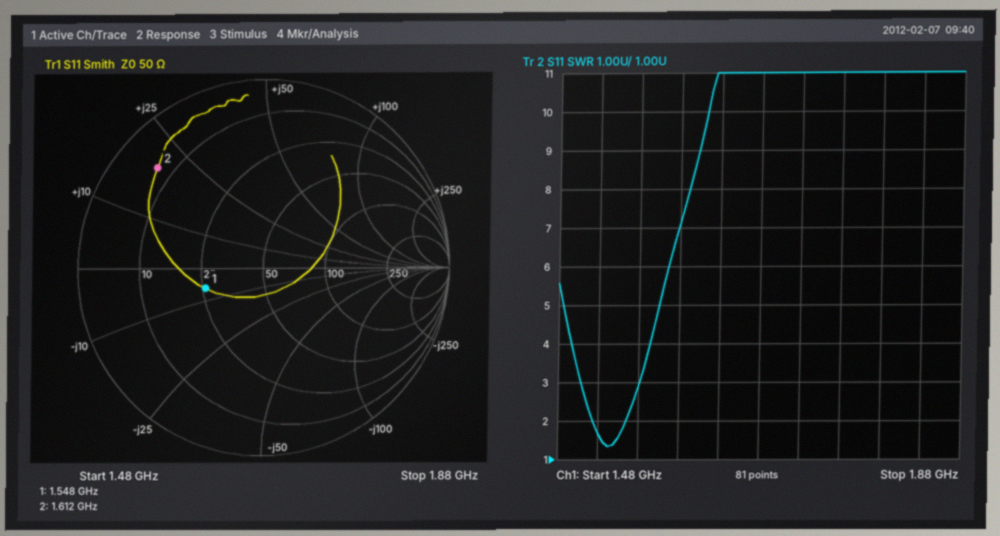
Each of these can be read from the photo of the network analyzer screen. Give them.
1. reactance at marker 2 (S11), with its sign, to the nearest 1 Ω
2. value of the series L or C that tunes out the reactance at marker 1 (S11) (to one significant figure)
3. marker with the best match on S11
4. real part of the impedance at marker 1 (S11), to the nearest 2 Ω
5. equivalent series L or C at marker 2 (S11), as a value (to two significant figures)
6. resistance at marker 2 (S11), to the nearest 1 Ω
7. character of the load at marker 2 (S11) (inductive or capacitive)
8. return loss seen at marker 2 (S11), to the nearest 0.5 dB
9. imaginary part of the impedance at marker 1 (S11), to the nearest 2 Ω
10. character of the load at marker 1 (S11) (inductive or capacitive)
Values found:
+19 Ω
600 pH
marker 1
26 Ω
1.9 nH
7 Ω
inductive
2.0 dB
-6 Ω
capacitive
